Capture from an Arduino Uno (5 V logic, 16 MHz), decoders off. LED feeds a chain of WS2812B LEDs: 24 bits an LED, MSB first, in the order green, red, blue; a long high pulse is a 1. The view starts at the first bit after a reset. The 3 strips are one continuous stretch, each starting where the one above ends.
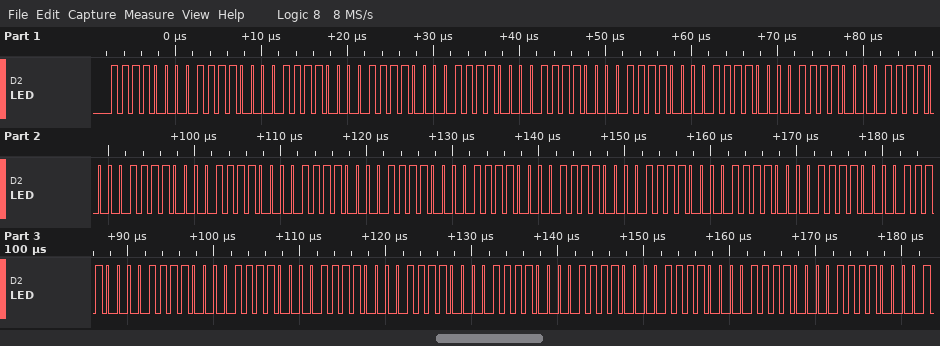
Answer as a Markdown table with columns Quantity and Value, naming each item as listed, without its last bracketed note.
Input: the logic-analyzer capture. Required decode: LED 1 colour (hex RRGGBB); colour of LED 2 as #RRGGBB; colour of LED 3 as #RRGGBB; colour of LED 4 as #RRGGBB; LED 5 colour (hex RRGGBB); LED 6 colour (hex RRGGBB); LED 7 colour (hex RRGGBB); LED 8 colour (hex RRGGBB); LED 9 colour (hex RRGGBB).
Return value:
| Quantity | Value |
|---|---|
| LED 1 colour | #F0F0F0 |
| colour of LED 2 as #RRGGBB | #F0F0F0 |
| colour of LED 3 as #RRGGBB | #F0F0F0 |
| colour of LED 4 as #RRGGBB | #F0F0F0 |
| LED 5 colour | #F0F0F0 |
| LED 6 colour | #F0F0F0 |
| LED 7 colour | #F0F0F0 |
| LED 8 colour | #F0F0F0 |
| LED 9 colour | #F0F0F0 |
